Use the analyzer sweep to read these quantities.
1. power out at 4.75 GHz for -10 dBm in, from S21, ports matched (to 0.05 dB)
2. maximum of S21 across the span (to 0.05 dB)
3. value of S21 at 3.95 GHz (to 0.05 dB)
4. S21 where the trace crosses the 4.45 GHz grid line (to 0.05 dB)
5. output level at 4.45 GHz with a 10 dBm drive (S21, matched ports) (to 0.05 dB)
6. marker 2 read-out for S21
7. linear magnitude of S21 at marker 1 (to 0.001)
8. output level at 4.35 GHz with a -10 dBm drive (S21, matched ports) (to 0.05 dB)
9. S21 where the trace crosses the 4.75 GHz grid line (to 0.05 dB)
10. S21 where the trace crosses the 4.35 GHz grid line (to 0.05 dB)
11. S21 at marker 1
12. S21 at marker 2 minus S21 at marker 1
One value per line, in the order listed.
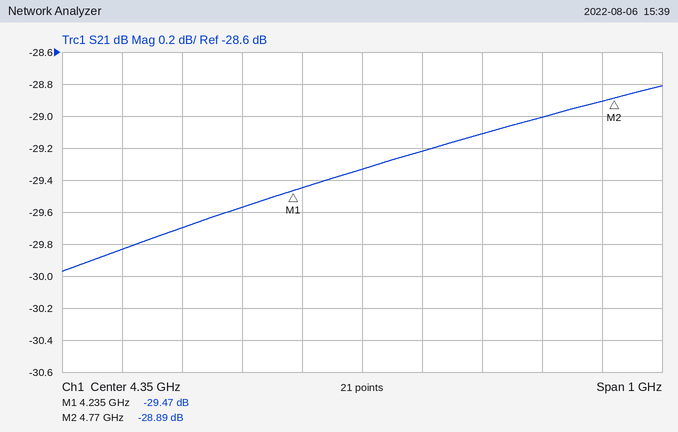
-38.90 dBm
-28.80 dB
-29.85 dB
-29.20 dB
-19.20 dBm
-28.89 dB
0.034
-39.35 dBm
-28.90 dB
-29.35 dB
-29.47 dB
0.58 dB
